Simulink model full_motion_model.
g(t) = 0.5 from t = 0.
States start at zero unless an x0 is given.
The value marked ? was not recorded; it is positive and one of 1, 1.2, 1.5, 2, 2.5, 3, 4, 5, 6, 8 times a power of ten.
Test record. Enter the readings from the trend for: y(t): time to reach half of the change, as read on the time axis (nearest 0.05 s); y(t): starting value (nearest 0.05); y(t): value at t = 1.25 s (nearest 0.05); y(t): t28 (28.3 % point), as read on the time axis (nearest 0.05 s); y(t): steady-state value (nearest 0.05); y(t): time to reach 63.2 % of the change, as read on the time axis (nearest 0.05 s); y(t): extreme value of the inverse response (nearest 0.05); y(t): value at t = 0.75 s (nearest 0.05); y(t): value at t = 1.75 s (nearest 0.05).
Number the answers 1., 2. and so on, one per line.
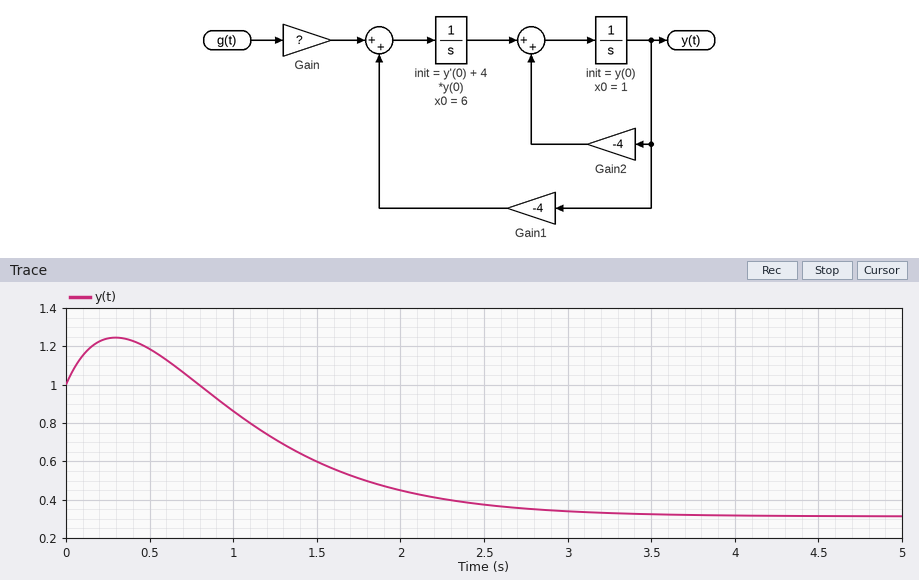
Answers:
1. 1.35 s
2. 1.00
3. 0.70
4. 1.10 s
5. 0.30
6. 1.60 s
7. 1.25
8. 1.05
9. 0.50
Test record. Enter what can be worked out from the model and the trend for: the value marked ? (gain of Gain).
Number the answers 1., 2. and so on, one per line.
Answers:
1. 2.5
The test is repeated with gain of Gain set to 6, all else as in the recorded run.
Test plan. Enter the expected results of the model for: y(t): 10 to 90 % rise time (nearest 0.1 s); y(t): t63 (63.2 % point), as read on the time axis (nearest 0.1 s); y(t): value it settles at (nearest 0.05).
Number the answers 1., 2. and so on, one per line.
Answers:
1. 1.4 s
2. 2.0 s
3. 0.75
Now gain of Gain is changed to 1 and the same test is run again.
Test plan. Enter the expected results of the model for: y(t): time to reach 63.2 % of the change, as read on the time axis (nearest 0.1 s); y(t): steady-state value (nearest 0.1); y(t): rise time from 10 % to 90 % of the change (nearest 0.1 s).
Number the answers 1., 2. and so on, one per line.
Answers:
1. 1.5 s
2. 0.1
3. 1.6 s
